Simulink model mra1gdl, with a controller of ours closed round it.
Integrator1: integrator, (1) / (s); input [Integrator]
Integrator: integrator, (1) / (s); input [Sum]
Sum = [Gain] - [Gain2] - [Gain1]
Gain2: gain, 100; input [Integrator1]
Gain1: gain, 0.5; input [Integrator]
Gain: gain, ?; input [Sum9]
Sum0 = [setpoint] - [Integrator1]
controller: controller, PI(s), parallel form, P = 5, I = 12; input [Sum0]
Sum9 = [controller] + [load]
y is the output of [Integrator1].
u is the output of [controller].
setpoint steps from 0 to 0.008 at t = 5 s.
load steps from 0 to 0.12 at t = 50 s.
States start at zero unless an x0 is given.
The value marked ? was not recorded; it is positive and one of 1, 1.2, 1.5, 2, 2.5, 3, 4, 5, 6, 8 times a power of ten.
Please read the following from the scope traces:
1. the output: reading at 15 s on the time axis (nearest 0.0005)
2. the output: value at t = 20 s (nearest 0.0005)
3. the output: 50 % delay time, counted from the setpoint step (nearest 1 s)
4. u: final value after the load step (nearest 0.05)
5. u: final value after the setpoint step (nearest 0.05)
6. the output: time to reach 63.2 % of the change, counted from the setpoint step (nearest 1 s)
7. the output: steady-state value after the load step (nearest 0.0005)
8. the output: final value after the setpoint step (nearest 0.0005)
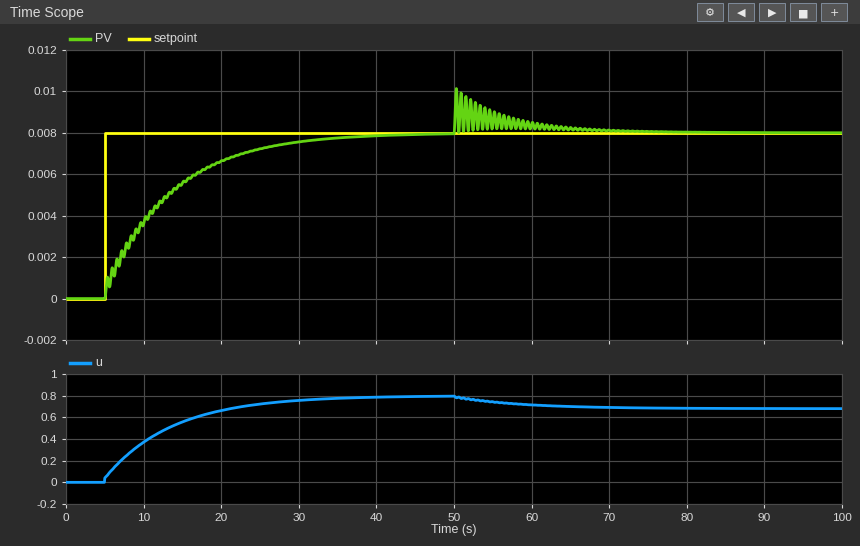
0.0055
0.0065
6 s
0.70
0.80
8 s
0.0080
0.0080
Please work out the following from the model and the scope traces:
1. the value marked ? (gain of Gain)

1
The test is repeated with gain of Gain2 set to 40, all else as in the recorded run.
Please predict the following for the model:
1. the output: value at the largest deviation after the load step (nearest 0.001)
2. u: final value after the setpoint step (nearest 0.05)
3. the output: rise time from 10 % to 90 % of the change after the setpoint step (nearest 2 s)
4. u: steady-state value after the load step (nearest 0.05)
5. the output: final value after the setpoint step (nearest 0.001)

0.013
0.30
6 s
0.20
0.008
